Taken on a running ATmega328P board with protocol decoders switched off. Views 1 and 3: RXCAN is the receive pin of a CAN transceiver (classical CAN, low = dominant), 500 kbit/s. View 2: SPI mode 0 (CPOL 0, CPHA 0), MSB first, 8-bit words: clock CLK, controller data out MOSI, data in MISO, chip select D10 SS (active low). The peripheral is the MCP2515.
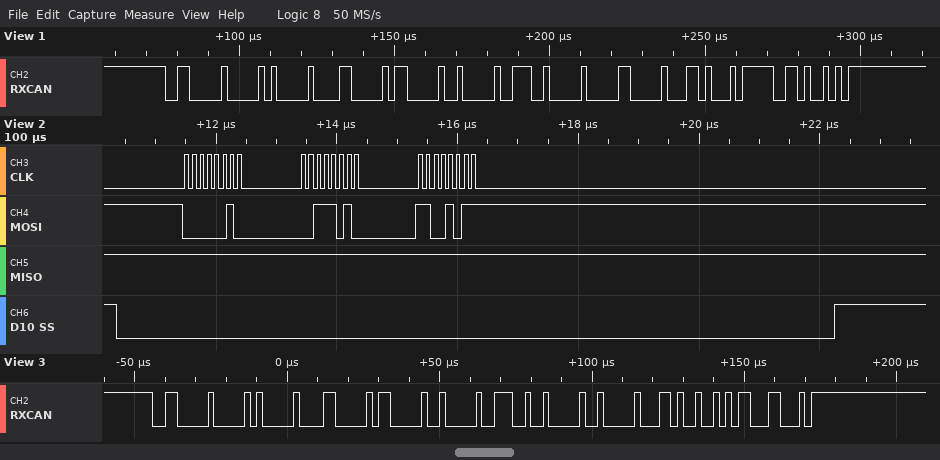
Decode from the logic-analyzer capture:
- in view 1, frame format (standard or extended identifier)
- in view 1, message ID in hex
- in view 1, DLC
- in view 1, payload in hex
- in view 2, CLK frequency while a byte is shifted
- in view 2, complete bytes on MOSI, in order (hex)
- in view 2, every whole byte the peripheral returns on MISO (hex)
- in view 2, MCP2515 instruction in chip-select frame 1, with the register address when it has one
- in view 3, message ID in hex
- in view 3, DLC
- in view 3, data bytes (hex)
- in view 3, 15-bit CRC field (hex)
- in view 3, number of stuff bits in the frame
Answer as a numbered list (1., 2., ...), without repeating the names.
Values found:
1. standard
2. 0x300
3. 8
4. 03 03 01 01 C8 01 00 D1
5. 8 MHz
6. 02 3A CB
7. FF FF FF
8. WRITE 0x3A
9. 0x300
10. 8
11. 03 03 01 01 C9 01 00 D2
12. 0x2B18
13. 8
